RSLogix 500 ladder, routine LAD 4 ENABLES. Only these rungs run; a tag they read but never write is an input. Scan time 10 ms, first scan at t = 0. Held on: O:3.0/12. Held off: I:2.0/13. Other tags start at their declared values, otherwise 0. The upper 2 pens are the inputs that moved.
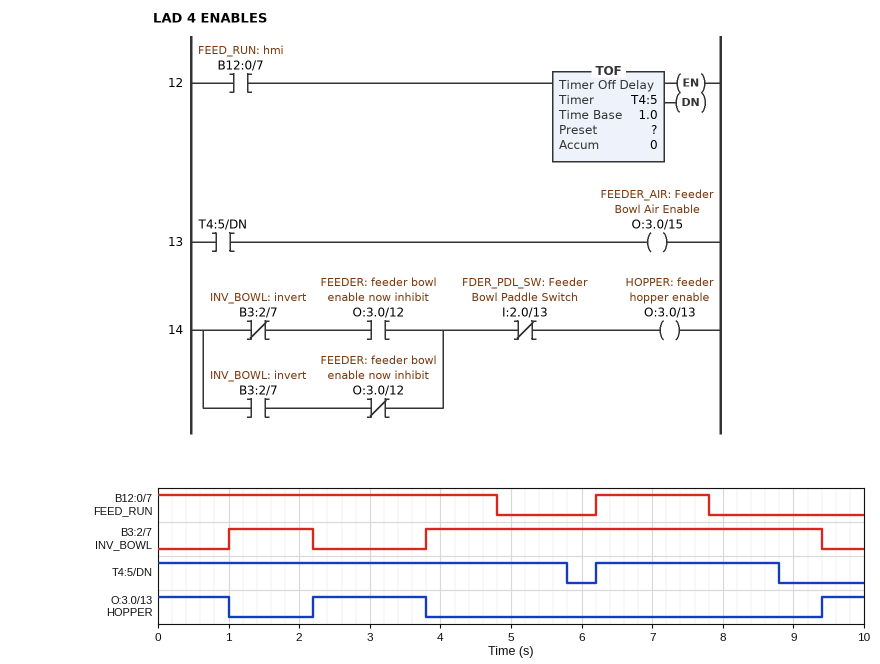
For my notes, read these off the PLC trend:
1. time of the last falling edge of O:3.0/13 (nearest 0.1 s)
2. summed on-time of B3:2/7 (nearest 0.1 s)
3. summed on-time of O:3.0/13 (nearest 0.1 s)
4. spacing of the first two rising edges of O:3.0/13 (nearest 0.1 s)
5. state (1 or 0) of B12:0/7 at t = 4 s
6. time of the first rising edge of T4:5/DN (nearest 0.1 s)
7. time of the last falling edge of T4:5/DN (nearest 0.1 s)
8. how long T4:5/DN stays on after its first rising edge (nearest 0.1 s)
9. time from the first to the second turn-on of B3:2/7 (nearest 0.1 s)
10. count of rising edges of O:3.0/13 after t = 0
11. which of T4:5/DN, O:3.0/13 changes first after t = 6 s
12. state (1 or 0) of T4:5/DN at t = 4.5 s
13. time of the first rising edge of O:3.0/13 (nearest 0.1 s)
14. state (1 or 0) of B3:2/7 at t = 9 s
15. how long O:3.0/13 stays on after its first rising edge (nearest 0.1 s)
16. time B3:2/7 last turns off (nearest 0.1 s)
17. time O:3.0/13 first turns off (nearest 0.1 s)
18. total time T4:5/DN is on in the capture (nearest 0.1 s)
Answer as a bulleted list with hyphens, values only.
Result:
- 3.8 s
- 6.8 s
- 3.2 s
- 7.2 s
- 1
- 6.2 s
- 8.8 s
- 2.6 s
- 2.8 s
- 2
- T4:5/DN
- 1
- 2.2 s
- 1
- 1.6 s
- 9.4 s
- 1.0 s
- 8.4 s
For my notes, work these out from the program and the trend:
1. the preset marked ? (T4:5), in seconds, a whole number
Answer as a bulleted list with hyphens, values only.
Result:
- 1 s
